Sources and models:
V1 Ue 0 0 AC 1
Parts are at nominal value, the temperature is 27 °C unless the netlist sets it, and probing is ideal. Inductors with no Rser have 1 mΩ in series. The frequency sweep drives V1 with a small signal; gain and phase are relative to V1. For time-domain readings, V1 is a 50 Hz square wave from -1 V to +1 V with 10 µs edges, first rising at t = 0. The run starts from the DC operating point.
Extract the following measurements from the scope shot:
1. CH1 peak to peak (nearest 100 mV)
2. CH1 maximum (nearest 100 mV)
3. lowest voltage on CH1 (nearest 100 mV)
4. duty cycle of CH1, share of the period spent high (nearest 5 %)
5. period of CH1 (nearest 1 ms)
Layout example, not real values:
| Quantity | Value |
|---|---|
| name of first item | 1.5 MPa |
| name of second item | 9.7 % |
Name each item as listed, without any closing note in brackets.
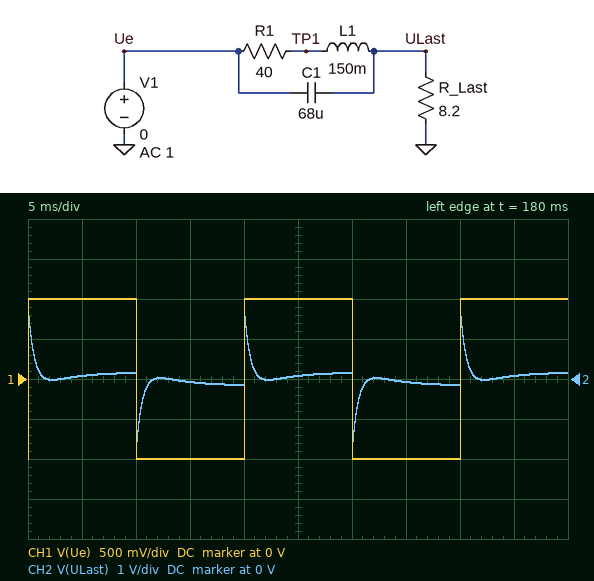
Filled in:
| Quantity | Value |
|---|---|
| CH1 peak to peak | 2.0 V |
| CH1 maximum | 1.0 V |
| lowest voltage on CH1 | -1.0 V |
| duty cycle of CH1, share of the period spent high | 50 % |
| period of CH1 | 20 ms |
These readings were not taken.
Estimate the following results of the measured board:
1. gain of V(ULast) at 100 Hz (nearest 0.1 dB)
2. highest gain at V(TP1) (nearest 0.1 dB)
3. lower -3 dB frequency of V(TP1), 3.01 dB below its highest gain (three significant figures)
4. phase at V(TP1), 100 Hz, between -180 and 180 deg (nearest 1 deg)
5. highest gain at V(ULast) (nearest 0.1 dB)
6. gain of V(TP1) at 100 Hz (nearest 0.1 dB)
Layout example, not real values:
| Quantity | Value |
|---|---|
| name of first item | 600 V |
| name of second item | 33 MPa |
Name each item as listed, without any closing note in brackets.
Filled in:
| Quantity | Value |
|---|---|
| gain of V(ULast) at 100 Hz | -11.7 dB |
| highest gain at V(TP1) | 0.6 dB |
| lower -3 dB frequency of V(TP1), 3.01 dB below its highest gain | 44.8 Hz |
| phase at V(TP1), 100 Hz, between -180 and 180 deg | 21 deg |
| highest gain at V(ULast) | 0 dB |
| gain of V(TP1) at 100 Hz | 0.1 dB |
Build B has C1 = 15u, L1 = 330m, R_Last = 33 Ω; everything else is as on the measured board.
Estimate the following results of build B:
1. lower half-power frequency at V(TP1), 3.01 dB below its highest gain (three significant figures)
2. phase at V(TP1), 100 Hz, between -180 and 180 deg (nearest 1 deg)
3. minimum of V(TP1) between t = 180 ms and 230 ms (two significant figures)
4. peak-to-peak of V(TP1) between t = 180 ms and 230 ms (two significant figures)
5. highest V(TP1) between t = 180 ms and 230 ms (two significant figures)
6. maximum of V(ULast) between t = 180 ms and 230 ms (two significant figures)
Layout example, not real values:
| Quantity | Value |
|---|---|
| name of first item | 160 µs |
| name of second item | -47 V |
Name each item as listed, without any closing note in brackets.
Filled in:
| Quantity | Value |
|---|---|
| lower half-power frequency at V(TP1), 3.01 dB below its highest gain | 27.5 Hz |
| phase at V(TP1), 100 Hz, between -180 and 180 deg | 10 deg |
| minimum of V(TP1) between t = 180 ms and 230 ms | -1.4 V |
| peak-to-peak of V(TP1) between t = 180 ms and 230 ms | 2.9 V |
| highest V(TP1) between t = 180 ms and 230 ms | 1.4 V |
| maximum of V(ULast) between t = 180 ms and 230 ms | 1.6 V |
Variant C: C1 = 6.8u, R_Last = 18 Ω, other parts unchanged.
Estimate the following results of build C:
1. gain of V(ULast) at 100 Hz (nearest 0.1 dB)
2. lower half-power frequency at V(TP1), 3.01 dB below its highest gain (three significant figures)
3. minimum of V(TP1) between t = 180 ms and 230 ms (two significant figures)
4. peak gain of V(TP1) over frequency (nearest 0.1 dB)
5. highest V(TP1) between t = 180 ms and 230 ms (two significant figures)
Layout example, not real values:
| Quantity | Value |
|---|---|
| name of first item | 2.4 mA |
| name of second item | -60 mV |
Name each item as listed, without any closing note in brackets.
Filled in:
| Quantity | Value |
|---|---|
| gain of V(ULast) at 100 Hz | -19.8 dB |
| lower half-power frequency at V(TP1), 3.01 dB below its highest gain | 55.3 Hz |
| minimum of V(TP1) between t = 180 ms and 230 ms | -1.7 V |
| peak gain of V(TP1) over frequency | 0.2 dB |
| highest V(TP1) between t = 180 ms and 230 ms | 1.7 V |
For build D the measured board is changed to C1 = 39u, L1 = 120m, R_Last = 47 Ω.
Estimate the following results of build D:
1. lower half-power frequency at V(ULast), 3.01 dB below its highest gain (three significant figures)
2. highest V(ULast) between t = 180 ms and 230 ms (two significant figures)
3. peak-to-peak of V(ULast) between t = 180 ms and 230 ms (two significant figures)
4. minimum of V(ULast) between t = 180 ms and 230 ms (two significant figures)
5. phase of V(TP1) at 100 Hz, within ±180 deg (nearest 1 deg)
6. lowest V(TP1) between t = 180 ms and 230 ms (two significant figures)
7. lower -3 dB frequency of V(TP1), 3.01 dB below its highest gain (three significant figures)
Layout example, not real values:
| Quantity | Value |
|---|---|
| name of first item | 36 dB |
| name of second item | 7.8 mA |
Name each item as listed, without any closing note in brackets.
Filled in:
| Quantity | Value |
|---|---|
| lower half-power frequency at V(ULast), 3.01 dB below its highest gain | 134 Hz |
| highest V(ULast) between t = 180 ms and 230 ms | 1.4 V |
| peak-to-peak of V(ULast) between t = 180 ms and 230 ms | 2.9 V |
| minimum of V(ULast) between t = 180 ms and 230 ms | -1.4 V |
| phase of V(TP1) at 100 Hz, within ±180 deg | 18 deg |
| lowest V(TP1) between t = 180 ms and 230 ms | -1.5 V |
| lower -3 dB frequency of V(TP1), 3.01 dB below its highest gain | 56.3 Hz |
